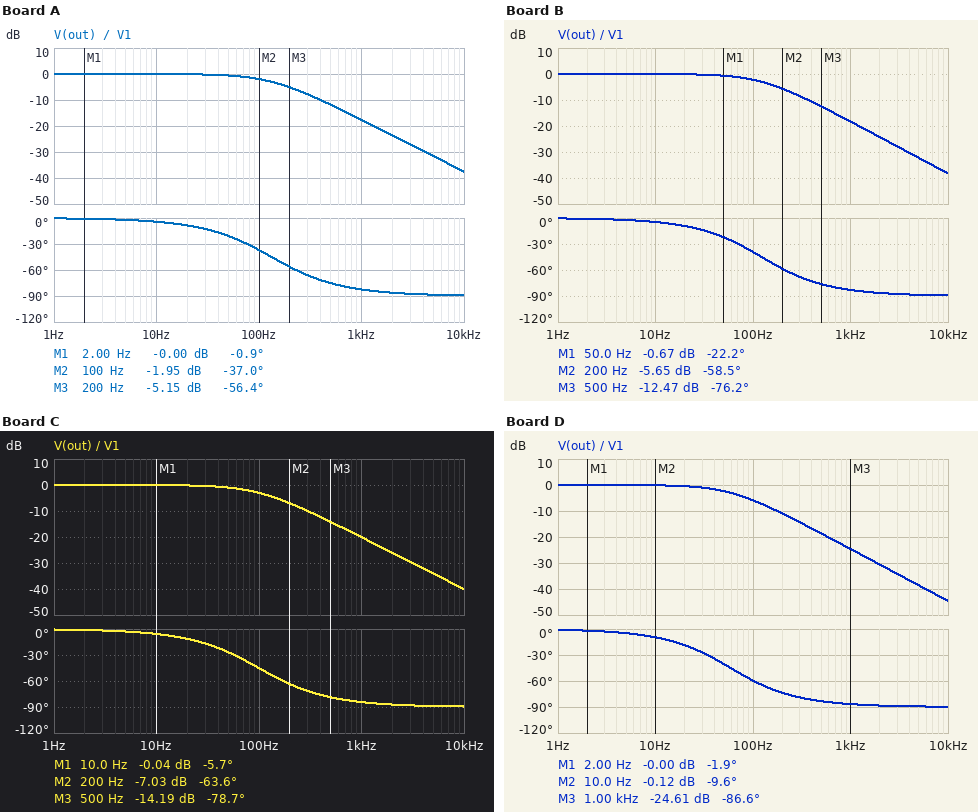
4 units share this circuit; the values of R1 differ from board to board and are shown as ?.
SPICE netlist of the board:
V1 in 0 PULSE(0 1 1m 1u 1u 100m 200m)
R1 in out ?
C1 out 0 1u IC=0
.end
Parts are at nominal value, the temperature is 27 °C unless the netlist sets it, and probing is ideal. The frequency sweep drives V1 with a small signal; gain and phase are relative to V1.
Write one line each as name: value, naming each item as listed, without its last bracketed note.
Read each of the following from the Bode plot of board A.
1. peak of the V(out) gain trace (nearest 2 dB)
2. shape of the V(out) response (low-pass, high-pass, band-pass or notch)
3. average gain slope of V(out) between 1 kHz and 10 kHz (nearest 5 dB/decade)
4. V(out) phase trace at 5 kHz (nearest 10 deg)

peak of the V(out) gain trace: 0 dB
shape of the V(out) response: low-pass
average gain slope of V(out) between 1 kHz and 10 kHz: -20 dB/decade
V(out) phase trace at 5 kHz: -90 deg
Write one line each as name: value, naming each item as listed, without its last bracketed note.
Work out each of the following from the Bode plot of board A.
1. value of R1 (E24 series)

value of R1: 1.2 kΩ
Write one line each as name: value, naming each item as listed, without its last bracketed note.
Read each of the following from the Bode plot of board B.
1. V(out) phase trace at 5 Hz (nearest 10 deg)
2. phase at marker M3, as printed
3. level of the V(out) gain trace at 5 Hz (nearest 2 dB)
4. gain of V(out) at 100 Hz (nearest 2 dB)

V(out) phase trace at 5 Hz: 0 deg
phase at marker M3, as printed: -76.2 deg
level of the V(out) gain trace at 5 Hz: 0 dB
gain of V(out) at 100 Hz: -2 dB
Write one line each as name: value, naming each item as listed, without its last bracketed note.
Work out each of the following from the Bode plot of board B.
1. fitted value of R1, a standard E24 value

fitted value of R1, a standard E24 value: 1.3 kΩ
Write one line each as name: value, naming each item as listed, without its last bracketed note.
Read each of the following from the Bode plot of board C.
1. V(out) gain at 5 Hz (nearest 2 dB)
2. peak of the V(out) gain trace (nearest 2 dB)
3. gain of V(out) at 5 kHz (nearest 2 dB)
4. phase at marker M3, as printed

V(out) gain at 5 Hz: 0 dB
peak of the V(out) gain trace: 0 dB
gain of V(out) at 5 kHz: -34 dB
phase at marker M3, as printed: -78.7 deg
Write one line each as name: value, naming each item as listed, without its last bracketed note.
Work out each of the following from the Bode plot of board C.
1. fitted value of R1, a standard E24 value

fitted value of R1, a standard E24 value: 1.6 kΩ
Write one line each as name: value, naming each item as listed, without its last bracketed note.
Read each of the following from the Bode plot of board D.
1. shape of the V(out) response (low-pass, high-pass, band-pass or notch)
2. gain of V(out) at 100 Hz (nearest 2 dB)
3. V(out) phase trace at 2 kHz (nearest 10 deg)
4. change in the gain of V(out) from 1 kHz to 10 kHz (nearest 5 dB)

shape of the V(out) response: low-pass
gain of V(out) at 100 Hz: -6 dB
V(out) phase trace at 2 kHz: -90 deg
change in the gain of V(out) from 1 kHz to 10 kHz: -20 dB
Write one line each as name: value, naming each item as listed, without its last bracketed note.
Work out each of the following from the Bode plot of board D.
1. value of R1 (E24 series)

value of R1: 2.7 kΩ
